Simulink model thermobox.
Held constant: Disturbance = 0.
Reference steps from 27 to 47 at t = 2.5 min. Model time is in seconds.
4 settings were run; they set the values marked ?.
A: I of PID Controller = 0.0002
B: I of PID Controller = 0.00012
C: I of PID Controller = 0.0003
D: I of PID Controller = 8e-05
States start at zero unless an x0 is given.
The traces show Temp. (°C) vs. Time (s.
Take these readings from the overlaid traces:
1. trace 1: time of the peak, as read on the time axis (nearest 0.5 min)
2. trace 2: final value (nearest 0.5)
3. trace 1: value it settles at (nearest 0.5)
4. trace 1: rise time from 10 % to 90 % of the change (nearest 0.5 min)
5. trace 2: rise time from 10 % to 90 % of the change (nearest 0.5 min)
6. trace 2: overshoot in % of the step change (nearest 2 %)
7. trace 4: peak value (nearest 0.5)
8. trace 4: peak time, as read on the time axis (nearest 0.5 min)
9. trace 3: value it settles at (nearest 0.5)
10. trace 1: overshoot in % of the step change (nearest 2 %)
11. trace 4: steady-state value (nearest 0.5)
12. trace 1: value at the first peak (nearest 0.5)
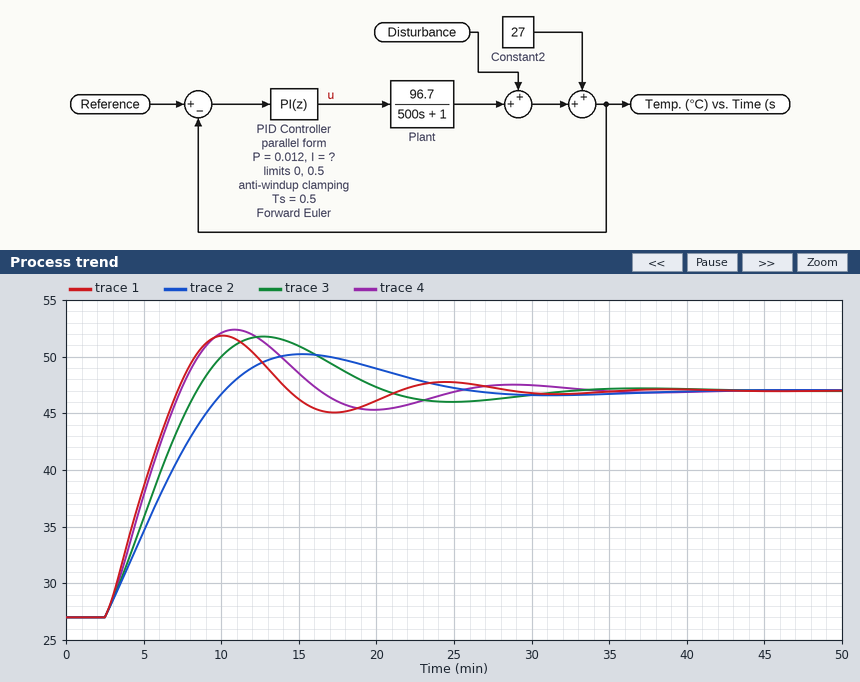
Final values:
10.0 min
47.0
47.0
3.5 min
6.0 min
16 %
52.5
11.0 min
47.0
24 %
47.0
52.0
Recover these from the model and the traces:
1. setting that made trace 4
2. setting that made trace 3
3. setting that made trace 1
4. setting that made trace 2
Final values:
A
B
C
D
